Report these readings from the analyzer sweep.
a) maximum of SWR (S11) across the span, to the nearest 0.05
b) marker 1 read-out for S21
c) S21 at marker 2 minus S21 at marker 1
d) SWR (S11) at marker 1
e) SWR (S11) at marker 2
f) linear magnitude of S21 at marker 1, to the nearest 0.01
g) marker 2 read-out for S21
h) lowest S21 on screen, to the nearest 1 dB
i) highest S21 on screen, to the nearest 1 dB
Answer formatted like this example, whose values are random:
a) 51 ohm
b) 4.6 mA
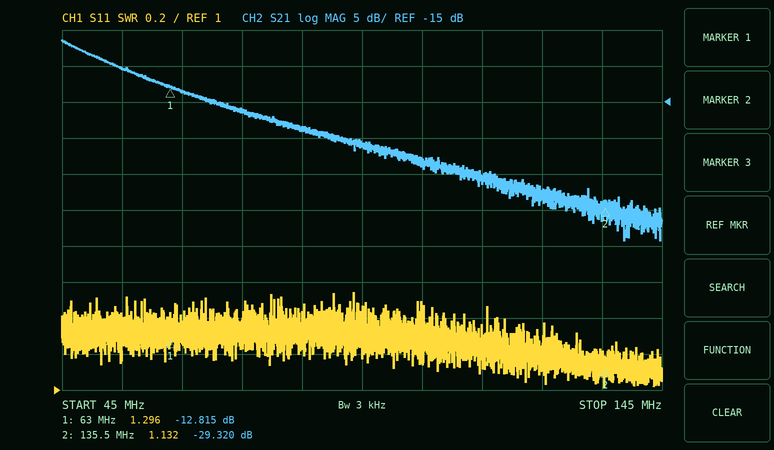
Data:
a) 1.55
b) -12.815 dB
c) -16.505 dB
d) 1.296
e) 1.132
f) 0.23
g) -29.320 dB
h) -34 dB
i) -6 dB
